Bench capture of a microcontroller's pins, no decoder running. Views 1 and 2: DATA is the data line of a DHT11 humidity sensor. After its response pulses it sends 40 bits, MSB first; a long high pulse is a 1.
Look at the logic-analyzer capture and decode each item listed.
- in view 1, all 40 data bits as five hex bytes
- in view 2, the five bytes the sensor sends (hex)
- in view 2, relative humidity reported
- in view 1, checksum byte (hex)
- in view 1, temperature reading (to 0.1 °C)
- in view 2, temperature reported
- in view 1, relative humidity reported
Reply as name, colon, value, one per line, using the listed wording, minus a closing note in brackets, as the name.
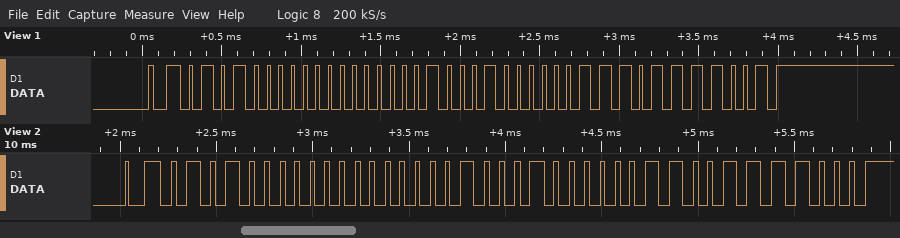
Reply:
in view 1, all 40 data bits as five hex bytes: 50 00 22 07 79
in view 2, the five bytes the sensor sends: 50 00 22 06 78
in view 2, relative humidity reported: 80 %
in view 1, checksum byte: 0x79
in view 1, temperature reading: 34.7 °C
in view 2, temperature reported: 34.6 °C
in view 1, relative humidity reported: 80 %
